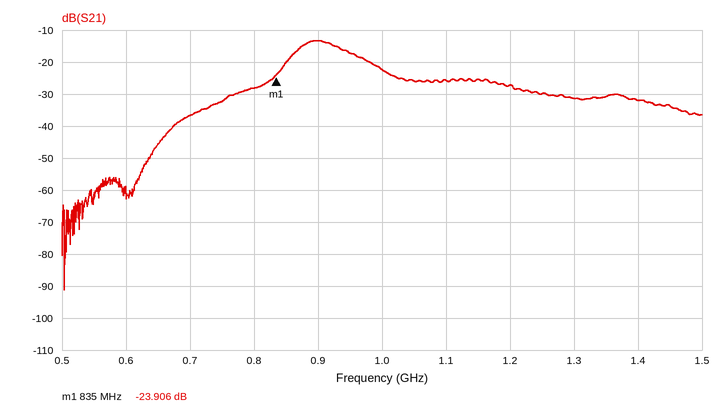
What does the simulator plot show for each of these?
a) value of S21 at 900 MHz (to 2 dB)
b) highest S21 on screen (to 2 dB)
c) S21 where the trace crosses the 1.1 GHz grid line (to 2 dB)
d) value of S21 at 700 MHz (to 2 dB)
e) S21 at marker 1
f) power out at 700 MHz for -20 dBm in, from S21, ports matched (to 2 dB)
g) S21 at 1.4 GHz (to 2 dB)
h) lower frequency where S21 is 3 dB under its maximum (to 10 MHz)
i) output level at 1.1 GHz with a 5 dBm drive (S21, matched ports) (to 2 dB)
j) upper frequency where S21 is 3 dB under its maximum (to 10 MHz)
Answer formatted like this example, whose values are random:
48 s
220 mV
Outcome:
-14 dB
-14 dB
-26 dB
-36 dB
-23.906 dB
-56 dBm
-32 dB
870 MHz
-20 dBm
940 MHz
